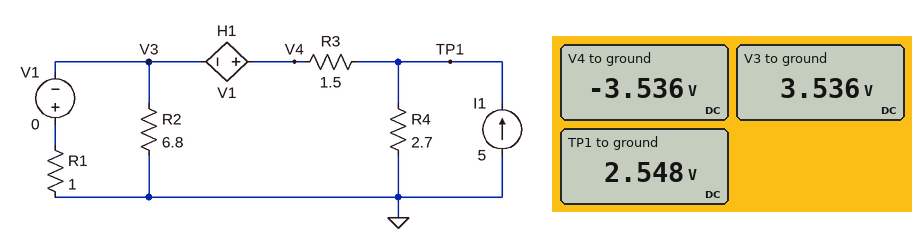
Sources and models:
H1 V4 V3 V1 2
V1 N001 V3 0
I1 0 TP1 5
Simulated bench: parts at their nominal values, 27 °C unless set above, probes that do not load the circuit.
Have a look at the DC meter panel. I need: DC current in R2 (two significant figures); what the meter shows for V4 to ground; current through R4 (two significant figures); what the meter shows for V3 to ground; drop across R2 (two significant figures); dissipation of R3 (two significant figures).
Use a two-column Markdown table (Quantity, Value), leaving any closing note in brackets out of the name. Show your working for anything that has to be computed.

| Quantity | Value |
|---|---|
| DC current in R2 | (3.536 V) / 6.8 Ω = 520 mA |
| what the meter shows for V4 to ground | -3.536 V |
| current through R4 | (2.548 V) / 2.7 Ω = 940 mA |
| what the meter shows for V3 to ground | 3.536 V |
| drop across R2 | 3.536 V = 3.5 V |
| dissipation of R3 | (2.548 V - (-3.536 V))^2 / 1.5 Ω = 25 W |
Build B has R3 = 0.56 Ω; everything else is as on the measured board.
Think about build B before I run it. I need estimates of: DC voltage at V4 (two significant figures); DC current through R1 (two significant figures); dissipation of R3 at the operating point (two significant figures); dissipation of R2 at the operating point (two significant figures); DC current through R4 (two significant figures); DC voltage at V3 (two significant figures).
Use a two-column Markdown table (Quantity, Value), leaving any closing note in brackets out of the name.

| Quantity | Value |
|---|---|
| DC voltage at V4 | -4.9 V |
| DC current through R1 | 4.9 A |
| dissipation of R3 at the operating point | 18 W |
| dissipation of R2 at the operating point | 3.6 W |
| DC current through R4 | 650 mA |
| DC voltage at V3 | 4.9 V |
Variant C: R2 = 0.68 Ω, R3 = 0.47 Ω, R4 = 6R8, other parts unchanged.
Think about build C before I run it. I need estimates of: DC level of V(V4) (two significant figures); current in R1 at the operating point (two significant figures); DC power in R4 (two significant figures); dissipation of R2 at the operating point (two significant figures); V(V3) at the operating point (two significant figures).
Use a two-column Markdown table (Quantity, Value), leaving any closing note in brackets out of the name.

| Quantity | Value |
|---|---|
| DC level of V(V4) | -2.0 V |
| current in R1 at the operating point | 2.0 A |
| DC power in R4 | 15 mW |
| dissipation of R2 at the operating point | 5.9 W |
| V(V3) at the operating point | 2.0 V |
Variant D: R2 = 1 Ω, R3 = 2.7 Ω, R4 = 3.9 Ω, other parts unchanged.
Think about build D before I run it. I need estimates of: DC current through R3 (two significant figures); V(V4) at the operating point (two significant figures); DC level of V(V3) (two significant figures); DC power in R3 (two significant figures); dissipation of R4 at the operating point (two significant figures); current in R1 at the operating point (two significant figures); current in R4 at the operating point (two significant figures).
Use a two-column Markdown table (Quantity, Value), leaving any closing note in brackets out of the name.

| Quantity | Value |
|---|---|
| DC current through R3 | 3.2 A |
| V(V4) at the operating point | -1.6 V |
| DC level of V(V3) | 1.6 V |
| DC power in R3 | 28 W |
| dissipation of R4 at the operating point | 13 W |
| current in R1 at the operating point | 1.6 A |
| current in R4 at the operating point | 1.8 A |
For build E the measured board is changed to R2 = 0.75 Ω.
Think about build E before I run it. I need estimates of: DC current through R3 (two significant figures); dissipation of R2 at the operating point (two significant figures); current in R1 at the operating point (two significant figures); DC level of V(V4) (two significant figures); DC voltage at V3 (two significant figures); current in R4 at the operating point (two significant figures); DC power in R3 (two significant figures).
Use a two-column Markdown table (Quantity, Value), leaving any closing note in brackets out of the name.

| Quantity | Value |
|---|---|
| DC current through R3 | 3.6 A |
| dissipation of R2 at the operating point | 3.1 W |
| current in R1 at the operating point | 1.5 A |
| DC level of V(V4) | -1.5 V |
| DC voltage at V3 | 1.5 V |
| current in R4 at the operating point | 1.4 A |
| DC power in R3 | 19 W |
